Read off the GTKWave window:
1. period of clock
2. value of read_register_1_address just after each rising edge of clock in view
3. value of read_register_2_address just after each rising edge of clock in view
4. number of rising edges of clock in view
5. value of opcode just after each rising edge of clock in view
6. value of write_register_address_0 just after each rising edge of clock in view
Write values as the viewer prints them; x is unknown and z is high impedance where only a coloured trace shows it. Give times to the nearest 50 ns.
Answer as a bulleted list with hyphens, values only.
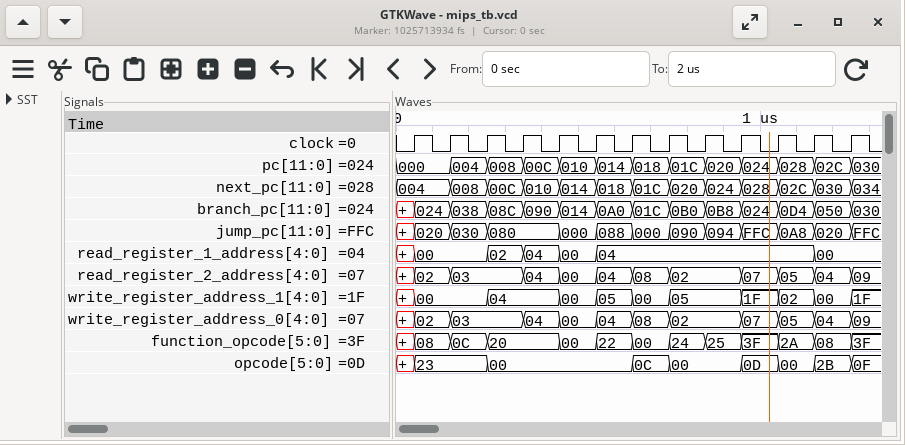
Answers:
- 100 ns
- 00, 00, 02, 04, 00, 04, 04, 04, 04, 04, 04, 00, 00
- 02, 03, 03, 04, 00, 04, 08, 02, 02, 07, 05, 04, 09
- 13
- 23, 23, 00, 00, 00, 00, 0C, 00, 00, 0D, 00, 2B, 0F
- 02, 03, 03, 04, 00, 04, 08, 02, 02, 07, 05, 04, 09
